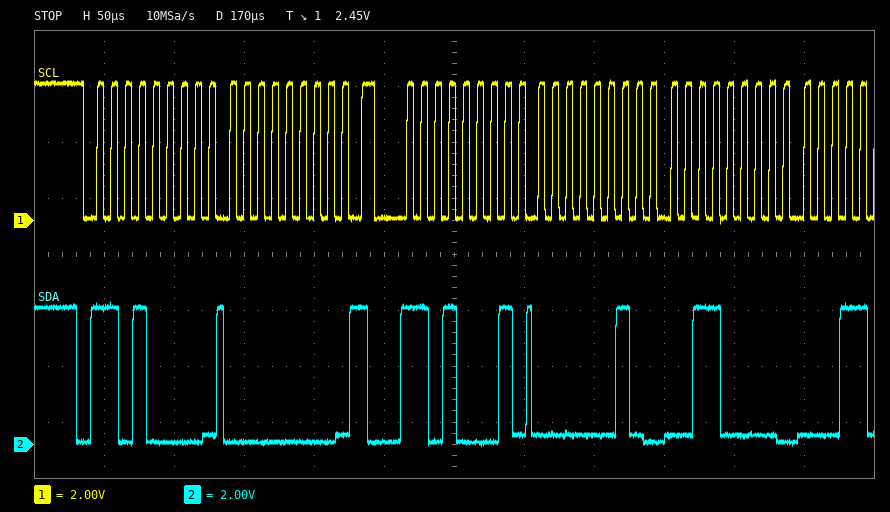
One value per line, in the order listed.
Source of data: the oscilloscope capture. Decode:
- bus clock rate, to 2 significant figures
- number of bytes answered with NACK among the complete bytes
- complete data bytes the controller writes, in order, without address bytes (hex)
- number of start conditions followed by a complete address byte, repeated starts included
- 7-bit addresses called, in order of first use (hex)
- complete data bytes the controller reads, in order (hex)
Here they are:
100 kHz
0
00
2
0x68
02 30
